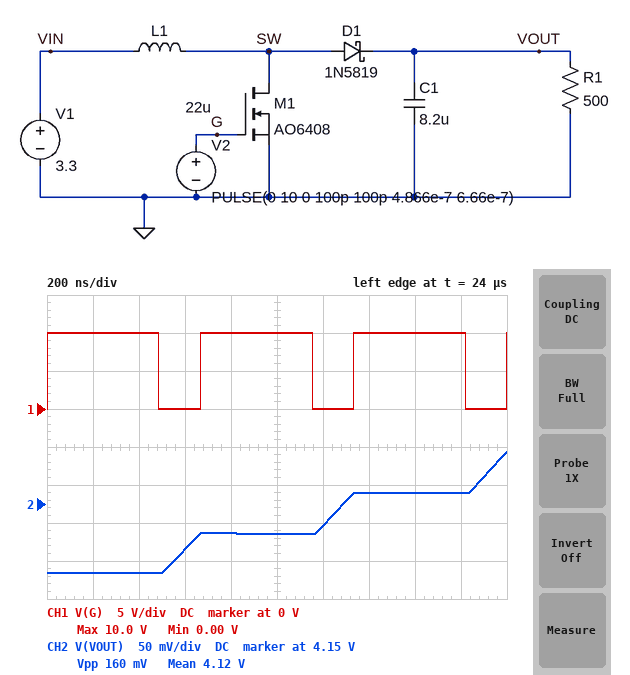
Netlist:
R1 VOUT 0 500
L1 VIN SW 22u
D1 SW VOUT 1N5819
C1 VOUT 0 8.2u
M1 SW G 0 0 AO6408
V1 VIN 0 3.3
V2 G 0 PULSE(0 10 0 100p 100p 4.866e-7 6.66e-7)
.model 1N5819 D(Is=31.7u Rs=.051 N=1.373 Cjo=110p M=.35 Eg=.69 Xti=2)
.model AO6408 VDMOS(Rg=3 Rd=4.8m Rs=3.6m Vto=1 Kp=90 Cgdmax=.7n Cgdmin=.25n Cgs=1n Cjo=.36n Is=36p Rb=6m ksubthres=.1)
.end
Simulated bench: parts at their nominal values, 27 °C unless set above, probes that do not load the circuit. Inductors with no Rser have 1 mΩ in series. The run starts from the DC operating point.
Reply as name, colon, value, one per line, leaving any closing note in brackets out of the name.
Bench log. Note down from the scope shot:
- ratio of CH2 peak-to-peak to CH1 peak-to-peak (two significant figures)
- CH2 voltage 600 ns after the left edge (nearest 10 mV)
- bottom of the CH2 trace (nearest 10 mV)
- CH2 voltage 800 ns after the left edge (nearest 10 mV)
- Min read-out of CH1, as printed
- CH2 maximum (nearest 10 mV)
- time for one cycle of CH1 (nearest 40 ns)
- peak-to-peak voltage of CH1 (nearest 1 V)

ratio of CH2 peak-to-peak to CH1 peak-to-peak: 0.016
CH2 voltage 600 ns after the left edge: 4.09 V
bottom of the CH2 trace: 4.06 V
CH2 voltage 800 ns after the left edge: 4.11 V
Min read-out of CH1, as printed: 0.00 V
CH2 maximum: 4.22 V
time for one cycle of CH1: 680 ns
peak-to-peak voltage of CH1: 10 V
